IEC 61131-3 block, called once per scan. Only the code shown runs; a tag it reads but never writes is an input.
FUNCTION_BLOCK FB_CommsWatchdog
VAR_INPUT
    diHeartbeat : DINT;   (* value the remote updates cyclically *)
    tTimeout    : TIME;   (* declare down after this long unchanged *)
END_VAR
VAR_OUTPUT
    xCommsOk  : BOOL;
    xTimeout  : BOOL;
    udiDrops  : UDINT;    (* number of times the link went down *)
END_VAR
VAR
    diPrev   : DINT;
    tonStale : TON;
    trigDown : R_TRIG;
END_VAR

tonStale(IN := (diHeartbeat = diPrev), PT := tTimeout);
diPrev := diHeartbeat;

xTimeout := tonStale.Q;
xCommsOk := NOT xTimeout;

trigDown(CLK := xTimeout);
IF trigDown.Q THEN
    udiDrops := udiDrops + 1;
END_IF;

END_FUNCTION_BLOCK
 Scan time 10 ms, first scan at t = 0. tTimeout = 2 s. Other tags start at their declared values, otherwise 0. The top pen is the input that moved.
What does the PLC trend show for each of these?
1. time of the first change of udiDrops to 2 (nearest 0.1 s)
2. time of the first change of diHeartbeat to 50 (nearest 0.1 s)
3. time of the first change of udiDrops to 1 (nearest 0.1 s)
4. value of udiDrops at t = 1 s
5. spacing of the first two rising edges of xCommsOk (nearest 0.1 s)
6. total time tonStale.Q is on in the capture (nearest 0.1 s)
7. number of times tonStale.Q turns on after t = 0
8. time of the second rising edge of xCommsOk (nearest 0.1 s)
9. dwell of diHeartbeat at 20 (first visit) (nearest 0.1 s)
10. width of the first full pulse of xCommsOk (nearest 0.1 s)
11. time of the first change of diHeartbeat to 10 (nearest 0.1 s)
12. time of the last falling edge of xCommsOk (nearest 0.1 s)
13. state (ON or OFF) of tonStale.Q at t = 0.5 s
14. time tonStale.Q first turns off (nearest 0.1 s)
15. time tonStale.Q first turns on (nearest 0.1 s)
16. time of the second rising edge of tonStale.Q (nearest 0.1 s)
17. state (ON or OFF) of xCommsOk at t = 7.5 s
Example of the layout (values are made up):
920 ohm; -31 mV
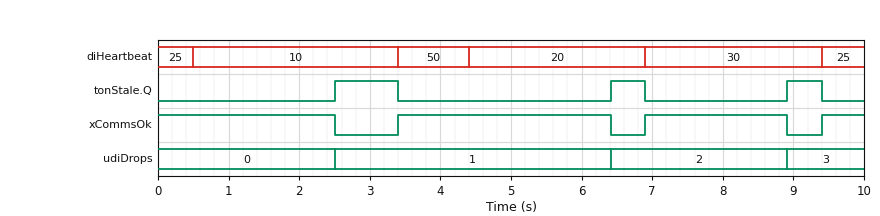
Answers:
6.4 s; 3.4 s; 2.5 s; 0; 3.5 s; 1.9 s; 3; 6.9 s; 2.5 s; 3.0 s; 0.5 s; 8.9 s; OFF; 3.4 s; 2.5 s; 6.4 s; ON
